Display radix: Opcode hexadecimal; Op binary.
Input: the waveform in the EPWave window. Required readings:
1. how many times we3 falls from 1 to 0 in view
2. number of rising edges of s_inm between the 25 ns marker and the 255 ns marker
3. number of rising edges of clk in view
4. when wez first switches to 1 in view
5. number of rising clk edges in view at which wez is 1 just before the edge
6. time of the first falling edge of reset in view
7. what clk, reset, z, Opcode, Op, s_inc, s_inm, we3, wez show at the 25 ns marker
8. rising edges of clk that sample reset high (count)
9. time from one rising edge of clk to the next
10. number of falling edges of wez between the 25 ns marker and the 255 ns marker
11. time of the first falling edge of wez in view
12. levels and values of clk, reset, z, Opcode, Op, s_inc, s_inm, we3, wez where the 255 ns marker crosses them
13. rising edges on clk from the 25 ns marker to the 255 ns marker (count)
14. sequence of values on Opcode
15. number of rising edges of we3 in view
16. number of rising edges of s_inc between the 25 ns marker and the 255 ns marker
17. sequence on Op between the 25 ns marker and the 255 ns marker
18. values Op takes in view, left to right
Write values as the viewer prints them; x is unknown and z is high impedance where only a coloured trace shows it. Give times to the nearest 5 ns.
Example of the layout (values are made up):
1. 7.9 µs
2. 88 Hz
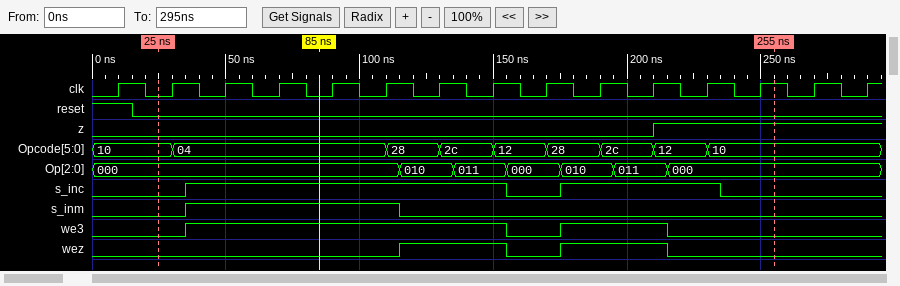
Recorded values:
1. 2
2. 1
3. 15
4. 115 ns
5. 4
6. 15 ns
7. clk=0, reset=0, z=0, Opcode=10, Op=000, s_inc=0, s_inm=0, we3=0, wez=0
8. 1
9. 20 ns
10. 2
11. 155 ns
12. clk=1, reset=0, z=1, Opcode=10, Op=000, s_inc=0, s_inm=0, we3=0, wez=0
13. 12
14. 10, 04, 28, 2c, 12, 28, 2c, 12, 10
15. 2
16. 2
17. 000, 010, 011, 000, 010, 011, 000
18. 000, 010, 011, 000, 010, 011, 000
